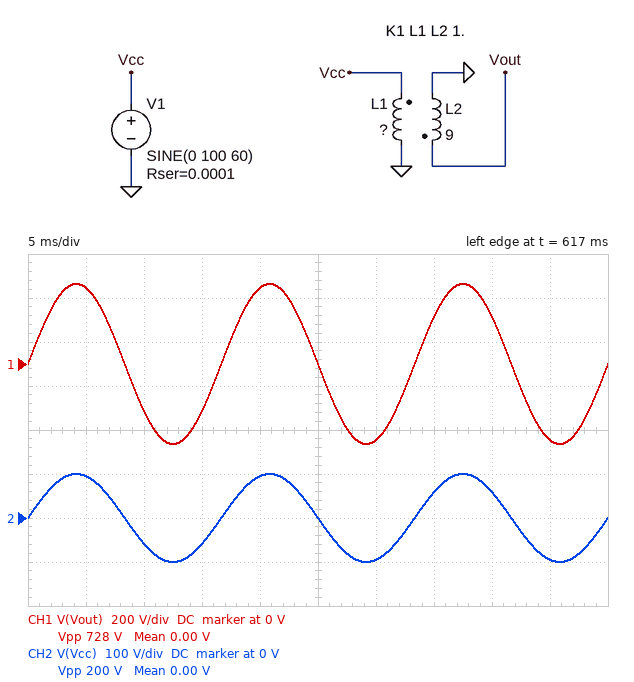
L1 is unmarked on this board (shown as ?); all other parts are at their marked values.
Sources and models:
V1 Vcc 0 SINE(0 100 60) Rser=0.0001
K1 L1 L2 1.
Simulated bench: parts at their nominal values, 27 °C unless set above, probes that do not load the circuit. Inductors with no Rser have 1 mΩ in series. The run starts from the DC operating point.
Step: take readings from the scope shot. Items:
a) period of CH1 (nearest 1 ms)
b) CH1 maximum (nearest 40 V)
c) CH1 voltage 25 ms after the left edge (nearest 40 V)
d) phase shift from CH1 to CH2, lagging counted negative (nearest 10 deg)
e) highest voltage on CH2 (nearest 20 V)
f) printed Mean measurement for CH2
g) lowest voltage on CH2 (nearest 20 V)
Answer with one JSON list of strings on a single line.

["17 ms", "360 V", "0 V", "0 deg", "100 V", "0.00 V", "-100 V"]
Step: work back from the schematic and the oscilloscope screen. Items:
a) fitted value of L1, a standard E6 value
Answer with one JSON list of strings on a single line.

["680 mH"]
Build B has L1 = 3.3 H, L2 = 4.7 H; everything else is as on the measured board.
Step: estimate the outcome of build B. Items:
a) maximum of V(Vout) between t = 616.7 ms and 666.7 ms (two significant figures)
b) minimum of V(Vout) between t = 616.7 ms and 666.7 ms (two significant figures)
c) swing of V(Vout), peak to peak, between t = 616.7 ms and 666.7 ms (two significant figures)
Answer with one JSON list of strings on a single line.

["120 V", "-120 V", "240 V"]
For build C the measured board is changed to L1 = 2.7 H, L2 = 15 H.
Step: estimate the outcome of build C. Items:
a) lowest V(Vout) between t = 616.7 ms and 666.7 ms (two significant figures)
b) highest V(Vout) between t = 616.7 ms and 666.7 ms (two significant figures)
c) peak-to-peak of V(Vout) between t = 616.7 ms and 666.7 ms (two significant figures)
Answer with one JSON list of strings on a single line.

["-240 V", "240 V", "470 V"]
